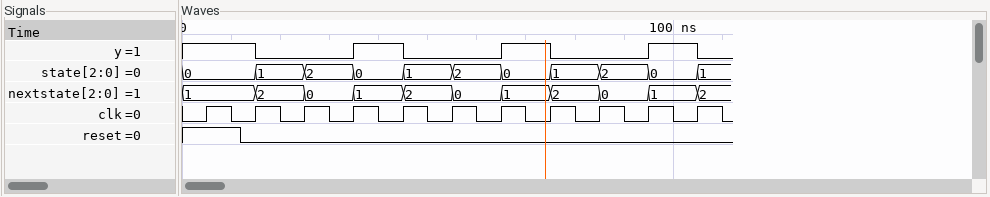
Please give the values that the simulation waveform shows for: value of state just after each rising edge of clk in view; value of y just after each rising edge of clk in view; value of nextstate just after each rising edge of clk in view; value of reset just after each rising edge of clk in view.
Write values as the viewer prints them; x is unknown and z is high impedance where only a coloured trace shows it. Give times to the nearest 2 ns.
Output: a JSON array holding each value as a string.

["0, 1, 2, 0, 1, 2, 0, 1, 2, 0, 1", "1 0 0 1 0 0 1 0 0 1 0", "1, 2, 0, 1, 2, 0, 1, 2, 0, 1, 2", "1 0 0 0 0 0 0 0 0 0 0"]
